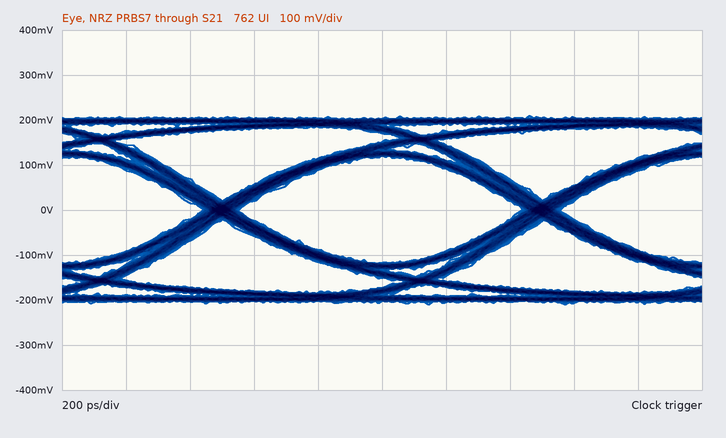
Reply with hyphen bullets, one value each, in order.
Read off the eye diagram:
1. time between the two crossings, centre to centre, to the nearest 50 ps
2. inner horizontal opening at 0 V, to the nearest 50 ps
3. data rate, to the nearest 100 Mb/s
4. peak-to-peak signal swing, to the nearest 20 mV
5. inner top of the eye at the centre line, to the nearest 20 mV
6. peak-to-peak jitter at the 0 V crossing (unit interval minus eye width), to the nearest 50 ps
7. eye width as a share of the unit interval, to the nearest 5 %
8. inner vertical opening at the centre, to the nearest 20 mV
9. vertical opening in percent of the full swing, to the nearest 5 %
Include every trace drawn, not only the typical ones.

- 1.00 ns
- 900 ps
- 1.0 Gb/s
- 420 mV
- 120 mV
- 100 ps
- 90 %
- 240 mV
- 55 %
